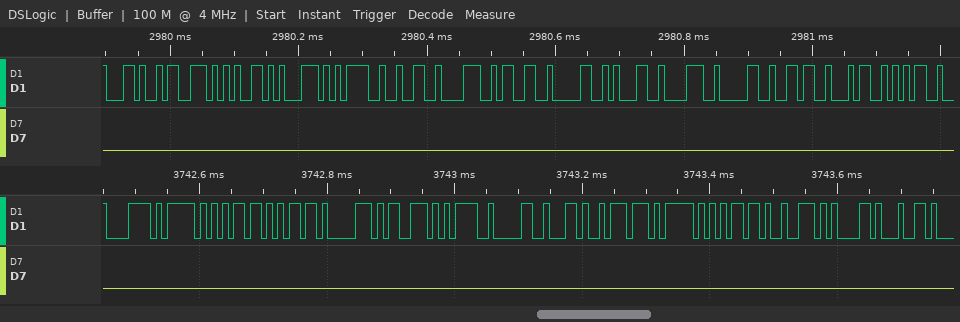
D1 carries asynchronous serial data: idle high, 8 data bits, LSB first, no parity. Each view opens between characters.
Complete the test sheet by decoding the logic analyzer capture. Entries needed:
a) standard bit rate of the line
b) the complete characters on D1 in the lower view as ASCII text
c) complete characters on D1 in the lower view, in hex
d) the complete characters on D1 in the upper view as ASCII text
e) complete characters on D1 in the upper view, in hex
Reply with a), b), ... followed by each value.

a) 115200 baud
b) "x_mmps=0,w_mrad"
c) 78, 5F, 6D, 6D, 70, 73, 3D, 30, 2C, 77, 5F, 6D, 72, 61, 64
d) ",seq=2830180645"
e) 2C, 73, 65, 71, 3D, 32, 38, 33, 30, 31, 38, 30, 36, 34, 35
